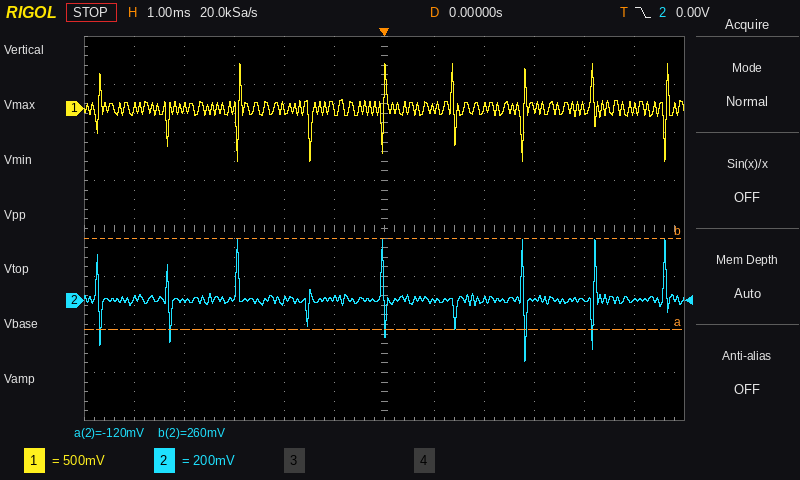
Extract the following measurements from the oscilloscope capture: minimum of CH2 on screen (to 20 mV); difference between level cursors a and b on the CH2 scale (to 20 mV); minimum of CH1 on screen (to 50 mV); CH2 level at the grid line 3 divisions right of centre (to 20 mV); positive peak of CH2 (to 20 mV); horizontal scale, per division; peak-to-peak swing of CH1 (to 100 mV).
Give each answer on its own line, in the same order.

-260 mV
380 mV
-550 mV
0 mV
260 mV
1 ms
1.00 V
